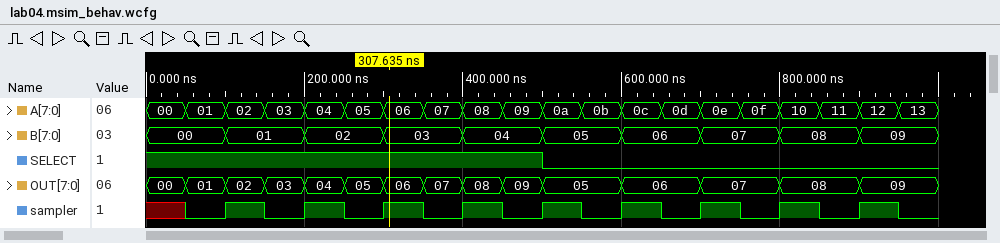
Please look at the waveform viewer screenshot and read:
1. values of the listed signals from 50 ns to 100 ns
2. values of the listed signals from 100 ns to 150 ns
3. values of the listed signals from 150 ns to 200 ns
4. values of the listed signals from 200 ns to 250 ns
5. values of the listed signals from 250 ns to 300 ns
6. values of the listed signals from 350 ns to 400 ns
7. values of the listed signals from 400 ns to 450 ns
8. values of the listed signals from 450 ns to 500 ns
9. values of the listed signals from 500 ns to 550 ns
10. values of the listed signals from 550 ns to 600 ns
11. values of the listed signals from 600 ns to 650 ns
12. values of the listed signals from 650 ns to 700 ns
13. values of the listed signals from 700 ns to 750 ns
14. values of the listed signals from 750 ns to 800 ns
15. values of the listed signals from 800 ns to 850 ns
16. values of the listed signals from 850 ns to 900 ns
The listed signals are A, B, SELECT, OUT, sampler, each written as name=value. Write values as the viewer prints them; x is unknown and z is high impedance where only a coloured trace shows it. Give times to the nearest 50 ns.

A=01, B=00, SELECT=1, OUT=01, sampler=0
A=02, B=01, SELECT=1, OUT=02, sampler=1
A=03, B=01, SELECT=1, OUT=03, sampler=0
A=04, B=02, SELECT=1, OUT=04, sampler=1
A=05, B=02, SELECT=1, OUT=05, sampler=0
A=07, B=03, SELECT=1, OUT=07, sampler=0
A=08, B=04, SELECT=1, OUT=08, sampler=1
A=09, B=04, SELECT=1, OUT=09, sampler=0
A=0a, B=05, SELECT=0, OUT=05, sampler=1
A=0b, B=05, SELECT=0, OUT=05, sampler=0
A=0c, B=06, SELECT=0, OUT=06, sampler=1
A=0d, B=06, SELECT=0, OUT=06, sampler=0
A=0e, B=07, SELECT=0, OUT=07, sampler=1
A=0f, B=07, SELECT=0, OUT=07, sampler=0
A=10, B=08, SELECT=0, OUT=08, sampler=1
A=11, B=08, SELECT=0, OUT=08, sampler=0
